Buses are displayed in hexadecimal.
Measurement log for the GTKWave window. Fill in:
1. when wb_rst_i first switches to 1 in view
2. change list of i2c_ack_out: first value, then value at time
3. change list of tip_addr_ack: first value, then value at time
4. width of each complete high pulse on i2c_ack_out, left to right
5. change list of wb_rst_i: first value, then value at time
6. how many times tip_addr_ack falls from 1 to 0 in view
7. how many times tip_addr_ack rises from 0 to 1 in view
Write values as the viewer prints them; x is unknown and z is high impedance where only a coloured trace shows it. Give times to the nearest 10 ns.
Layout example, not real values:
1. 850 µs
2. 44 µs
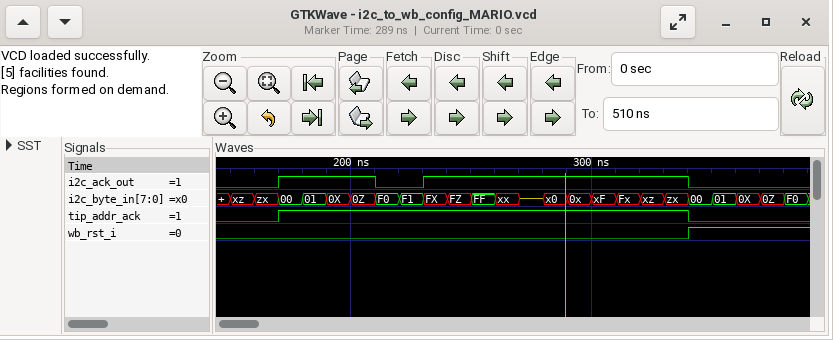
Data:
1. 340 ns
2. 0, 1 at 170 ns, 0 at 210 ns, 1 at 230 ns, 0 at 340 ns
3. 0, 1 at 170 ns, 0 at 340 ns
4. 40 ns, 110 ns
5. 0, 1 at 340 ns
6. 1
7. 1
